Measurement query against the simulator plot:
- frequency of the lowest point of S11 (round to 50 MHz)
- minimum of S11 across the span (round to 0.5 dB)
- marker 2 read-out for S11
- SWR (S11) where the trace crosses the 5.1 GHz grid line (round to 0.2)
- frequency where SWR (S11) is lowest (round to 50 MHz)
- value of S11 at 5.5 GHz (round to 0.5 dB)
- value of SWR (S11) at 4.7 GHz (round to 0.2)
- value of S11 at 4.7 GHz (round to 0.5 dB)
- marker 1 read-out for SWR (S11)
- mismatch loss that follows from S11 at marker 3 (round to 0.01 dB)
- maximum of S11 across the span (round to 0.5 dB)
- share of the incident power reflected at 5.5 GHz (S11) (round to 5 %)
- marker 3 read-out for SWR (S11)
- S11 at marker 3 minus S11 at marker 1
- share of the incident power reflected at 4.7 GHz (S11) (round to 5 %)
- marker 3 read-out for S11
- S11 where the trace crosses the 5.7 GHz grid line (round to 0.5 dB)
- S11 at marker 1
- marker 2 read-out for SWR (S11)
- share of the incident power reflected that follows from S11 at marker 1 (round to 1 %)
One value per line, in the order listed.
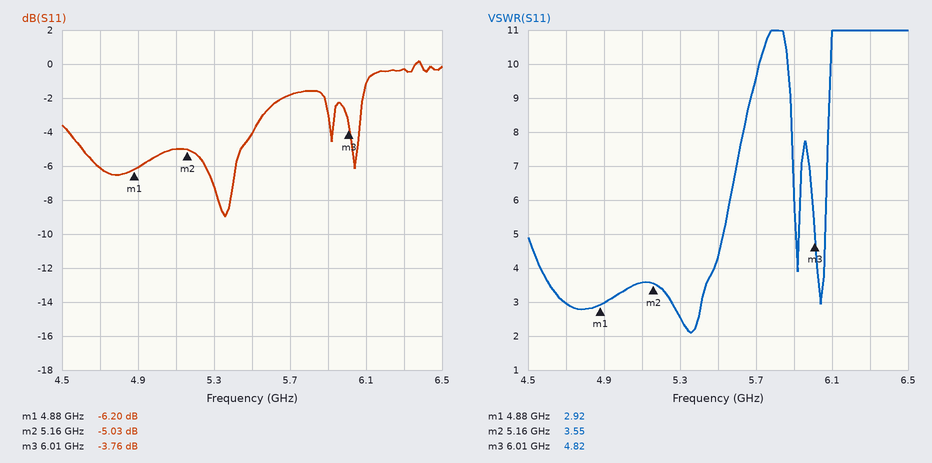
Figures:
5.35 GHz
-9.0 dB
-5.03 dB
3.6
5.35 GHz
-4.0 dB
3.0
-6.0 dB
2.92
2.37 dB
0.0 dB
40 %
4.82
2.44 dB
25 %
-3.76 dB
-2.0 dB
-6.20 dB
3.55
24 %
